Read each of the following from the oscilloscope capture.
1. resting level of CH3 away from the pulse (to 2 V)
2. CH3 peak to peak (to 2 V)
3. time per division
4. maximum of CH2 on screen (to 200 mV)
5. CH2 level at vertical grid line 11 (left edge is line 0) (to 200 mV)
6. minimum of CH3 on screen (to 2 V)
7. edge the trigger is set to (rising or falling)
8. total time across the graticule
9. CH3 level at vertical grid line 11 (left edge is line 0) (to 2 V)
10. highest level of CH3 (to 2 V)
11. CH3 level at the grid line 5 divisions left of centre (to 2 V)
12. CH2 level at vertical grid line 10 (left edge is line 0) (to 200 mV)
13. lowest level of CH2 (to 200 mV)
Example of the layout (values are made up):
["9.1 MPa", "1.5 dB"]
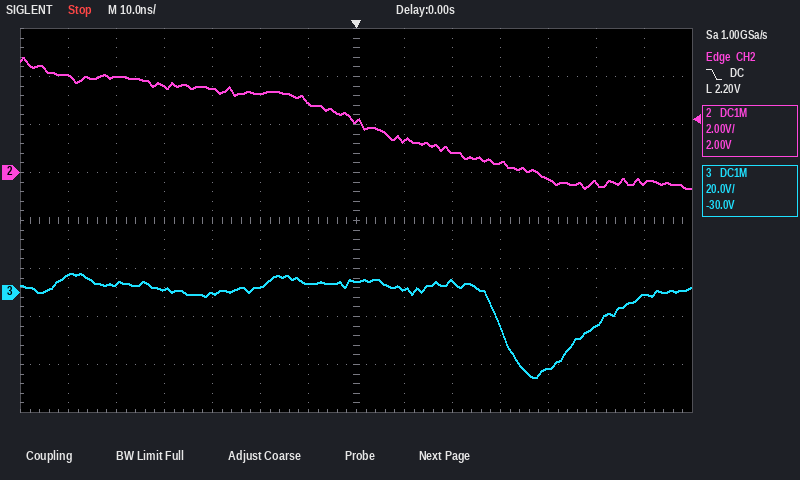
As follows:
["2 V", "44 V", "10 ns", "4.8 V", "-200 mV", "-36 V", "falling", "140 ns", "-32 V", "8 V", "4 V", "400 mV", "-600 mV"]
